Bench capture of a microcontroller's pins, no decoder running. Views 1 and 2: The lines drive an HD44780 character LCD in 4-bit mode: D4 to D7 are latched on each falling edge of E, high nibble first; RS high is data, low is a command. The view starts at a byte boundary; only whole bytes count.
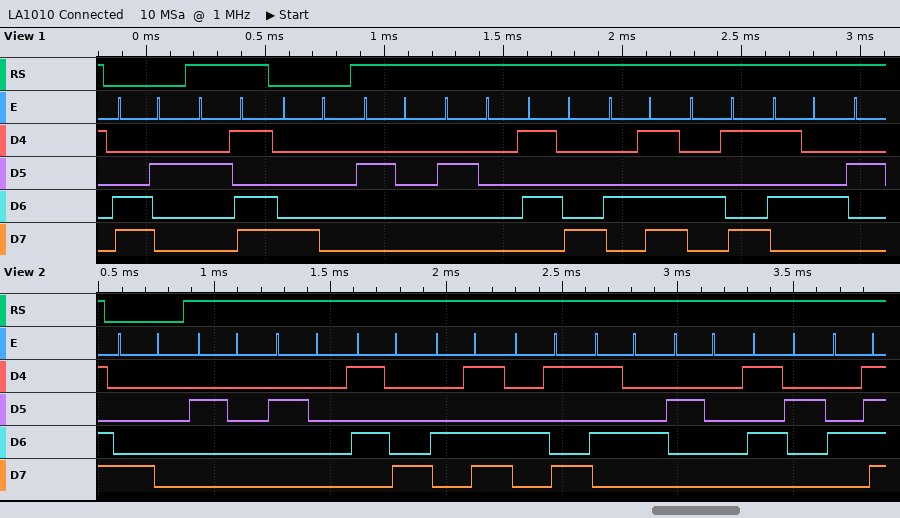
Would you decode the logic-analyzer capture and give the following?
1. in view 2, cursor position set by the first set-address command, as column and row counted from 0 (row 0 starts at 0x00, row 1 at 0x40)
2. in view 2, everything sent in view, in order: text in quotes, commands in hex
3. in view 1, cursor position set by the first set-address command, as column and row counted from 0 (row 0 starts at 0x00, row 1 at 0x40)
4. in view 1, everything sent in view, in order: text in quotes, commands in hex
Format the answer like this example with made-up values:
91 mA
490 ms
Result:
column 0, row 0
0x80 "  XMIT RO"
column 2, row 1
0xC2 "-" 0x80 "  XMIT"
